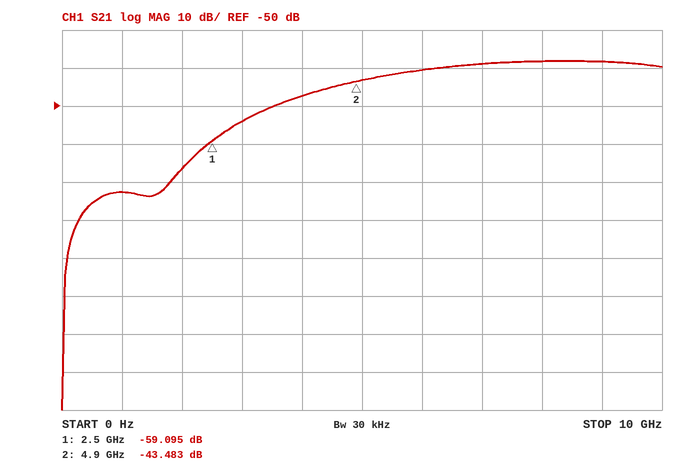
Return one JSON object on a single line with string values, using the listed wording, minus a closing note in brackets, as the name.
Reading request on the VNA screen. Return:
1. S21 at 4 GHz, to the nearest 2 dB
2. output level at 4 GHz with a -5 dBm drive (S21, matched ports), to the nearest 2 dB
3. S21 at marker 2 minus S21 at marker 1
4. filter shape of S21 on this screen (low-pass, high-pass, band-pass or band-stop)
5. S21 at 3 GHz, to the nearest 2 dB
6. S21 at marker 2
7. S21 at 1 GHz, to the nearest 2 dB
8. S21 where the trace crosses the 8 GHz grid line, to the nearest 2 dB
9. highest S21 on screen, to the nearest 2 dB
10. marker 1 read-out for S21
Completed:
{"S21 at 4 GHz, to the nearest 2 dB": "-48 dB", "output level at 4 GHz with a -5 dBm drive (S21, matched ports), to the nearest 2 dB": "-52 dBm", "S21 at marker 2 minus S21 at marker 1": "15.612 dB", "filter shape of S21 on this screen": "high-pass", "S21 at 3 GHz, to the nearest 2 dB": "-54 dB", "S21 at marker 2": "-43.483 dB", "S21 at 1 GHz, to the nearest 2 dB": "-72 dB", "S21 where the trace crosses the 8 GHz grid line, to the nearest 2 dB": "-38 dB", "highest S21 on screen, to the nearest 2 dB": "-38 dB", "marker 1 read-out for S21": "-59.095 dB"}
